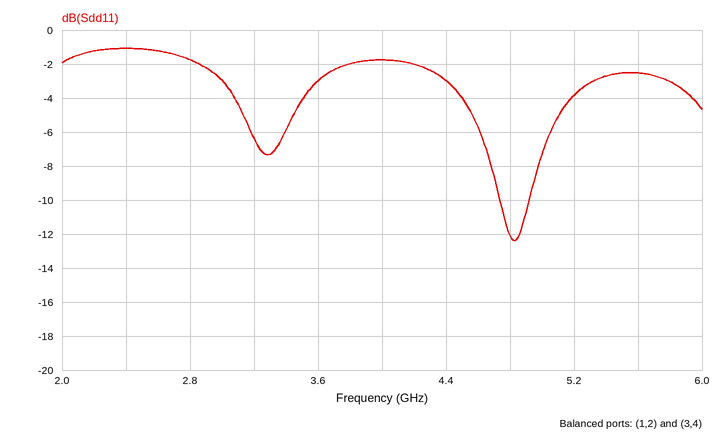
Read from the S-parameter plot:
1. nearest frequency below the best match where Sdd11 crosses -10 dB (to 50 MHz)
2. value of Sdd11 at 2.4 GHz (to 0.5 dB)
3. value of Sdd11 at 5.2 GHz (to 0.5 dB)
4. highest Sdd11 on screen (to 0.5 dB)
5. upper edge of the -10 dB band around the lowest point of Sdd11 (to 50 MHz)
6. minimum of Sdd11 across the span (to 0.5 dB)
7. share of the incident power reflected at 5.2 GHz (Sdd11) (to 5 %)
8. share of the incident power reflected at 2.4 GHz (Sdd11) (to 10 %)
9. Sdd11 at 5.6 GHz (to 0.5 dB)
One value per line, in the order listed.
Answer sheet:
4.75 GHz
-1.0 dB
-4.0 dB
-1.0 dB
4.90 GHz
-12.5 dB
40 %
80 %
-2.5 dB
